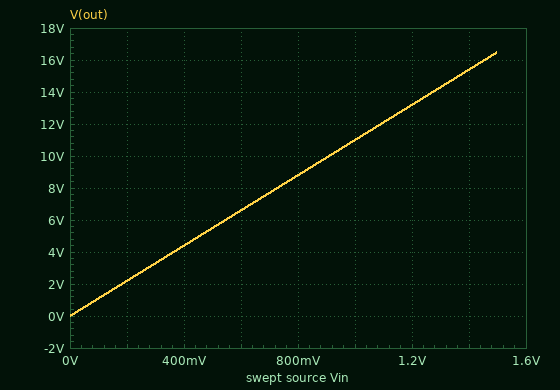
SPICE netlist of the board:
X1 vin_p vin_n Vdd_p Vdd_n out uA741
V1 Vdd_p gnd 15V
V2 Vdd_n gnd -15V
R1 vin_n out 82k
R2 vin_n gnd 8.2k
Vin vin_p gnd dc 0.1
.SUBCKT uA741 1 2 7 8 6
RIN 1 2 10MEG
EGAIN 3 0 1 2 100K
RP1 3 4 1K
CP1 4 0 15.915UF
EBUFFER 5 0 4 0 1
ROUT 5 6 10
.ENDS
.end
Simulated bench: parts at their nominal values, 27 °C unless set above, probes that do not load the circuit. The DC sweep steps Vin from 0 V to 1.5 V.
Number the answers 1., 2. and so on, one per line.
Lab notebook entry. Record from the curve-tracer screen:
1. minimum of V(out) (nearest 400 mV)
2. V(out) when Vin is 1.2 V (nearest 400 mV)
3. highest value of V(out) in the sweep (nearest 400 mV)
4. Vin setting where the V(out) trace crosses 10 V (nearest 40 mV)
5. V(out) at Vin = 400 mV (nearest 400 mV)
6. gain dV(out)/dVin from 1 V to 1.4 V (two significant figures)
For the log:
1. 0 V
2. 13.2 V
3. 16.4 V
4. 920 mV
5. 4.4 V
6. 11 V/V
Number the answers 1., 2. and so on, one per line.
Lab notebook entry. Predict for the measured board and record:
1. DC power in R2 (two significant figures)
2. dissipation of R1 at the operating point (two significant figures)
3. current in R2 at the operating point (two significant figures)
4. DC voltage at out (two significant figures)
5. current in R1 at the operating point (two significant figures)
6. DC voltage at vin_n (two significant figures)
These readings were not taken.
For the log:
1. 1.2 µW
2. 12 µW
3. 12 µA
4. 1.1 V
5. 12 µA
6. 100 mV
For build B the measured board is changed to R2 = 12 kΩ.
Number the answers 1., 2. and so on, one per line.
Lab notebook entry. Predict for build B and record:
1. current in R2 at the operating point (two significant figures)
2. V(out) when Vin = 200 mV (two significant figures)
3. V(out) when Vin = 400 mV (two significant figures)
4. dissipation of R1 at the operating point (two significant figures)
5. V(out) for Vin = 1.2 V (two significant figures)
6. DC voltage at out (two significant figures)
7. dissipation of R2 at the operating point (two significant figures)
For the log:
1. 8.3 µA
2. 1.6 V
3. 3.1 V
4. 5.7 µW
5. 9.4 V
6. 780 mV
7. 830 nW
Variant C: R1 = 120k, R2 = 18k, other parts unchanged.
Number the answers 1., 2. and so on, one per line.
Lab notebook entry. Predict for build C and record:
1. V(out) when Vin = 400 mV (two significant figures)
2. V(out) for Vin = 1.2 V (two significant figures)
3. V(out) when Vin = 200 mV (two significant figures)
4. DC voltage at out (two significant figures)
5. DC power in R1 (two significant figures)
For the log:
1. 3.1 V
2. 9.2 V
3. 1.5 V
4. 770 mV
5. 3.7 µW
